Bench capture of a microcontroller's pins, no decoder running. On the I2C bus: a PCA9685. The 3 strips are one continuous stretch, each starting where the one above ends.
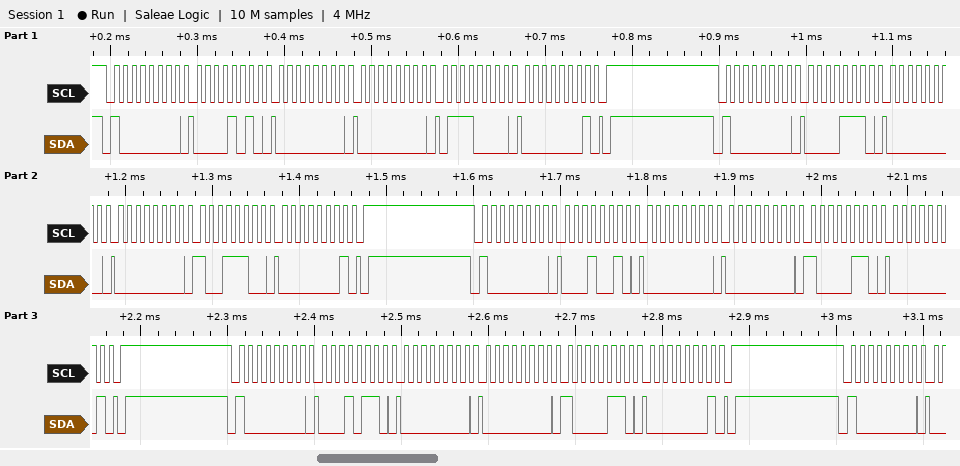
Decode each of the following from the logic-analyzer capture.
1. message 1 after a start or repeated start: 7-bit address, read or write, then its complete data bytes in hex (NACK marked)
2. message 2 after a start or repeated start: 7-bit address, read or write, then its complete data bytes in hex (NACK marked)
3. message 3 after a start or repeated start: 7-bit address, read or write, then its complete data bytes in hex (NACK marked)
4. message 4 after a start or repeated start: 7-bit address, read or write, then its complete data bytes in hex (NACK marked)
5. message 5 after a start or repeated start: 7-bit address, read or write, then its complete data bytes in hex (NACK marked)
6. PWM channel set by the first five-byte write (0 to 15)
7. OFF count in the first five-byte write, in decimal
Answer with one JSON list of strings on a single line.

["0x40 write: 0A 00 00 70 01", "0x40 write: 0E 00 00 9C 01", "0x40 write: 12 00 00 86 01", "0x40 write: 16 00 00 86 01", "0x40 write", "1", "368"]
